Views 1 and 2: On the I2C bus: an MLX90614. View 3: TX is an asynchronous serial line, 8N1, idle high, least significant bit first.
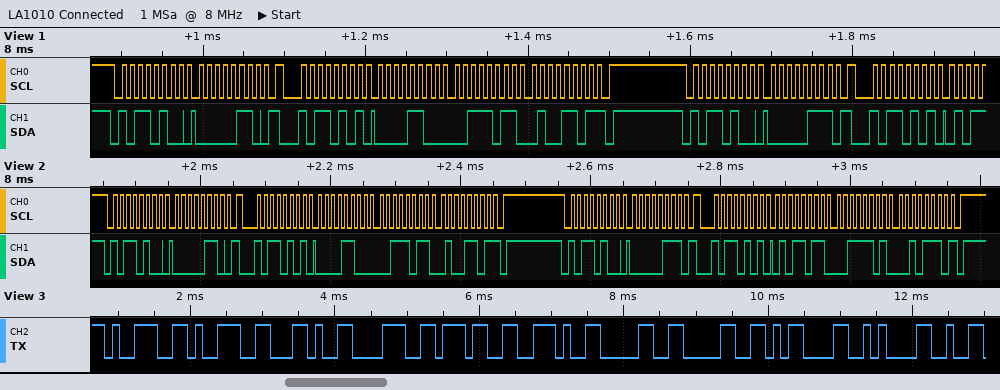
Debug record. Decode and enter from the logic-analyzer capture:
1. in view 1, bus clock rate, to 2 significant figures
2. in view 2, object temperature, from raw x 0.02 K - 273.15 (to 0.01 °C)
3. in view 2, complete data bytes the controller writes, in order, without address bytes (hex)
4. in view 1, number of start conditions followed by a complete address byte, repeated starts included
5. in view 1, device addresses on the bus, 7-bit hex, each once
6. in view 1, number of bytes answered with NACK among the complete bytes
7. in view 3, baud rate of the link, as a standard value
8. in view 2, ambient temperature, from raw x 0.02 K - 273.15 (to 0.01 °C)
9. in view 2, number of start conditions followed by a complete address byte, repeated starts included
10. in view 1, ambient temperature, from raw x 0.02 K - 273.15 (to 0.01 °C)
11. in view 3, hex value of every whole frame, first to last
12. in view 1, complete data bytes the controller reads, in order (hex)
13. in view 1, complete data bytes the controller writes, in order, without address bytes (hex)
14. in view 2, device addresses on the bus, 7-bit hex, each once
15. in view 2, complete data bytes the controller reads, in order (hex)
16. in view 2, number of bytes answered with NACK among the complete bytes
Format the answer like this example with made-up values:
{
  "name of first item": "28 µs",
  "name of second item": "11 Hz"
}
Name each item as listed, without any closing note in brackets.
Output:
{
  "in view 1, bus clock rate, to 2 significant figures": "100 kHz",
  "in view 2, object temperature, from raw x 0.02 K - 273.15": "40.99 °C",
  "in view 2, complete data bytes the controller writes, in order, without address bytes": "06 07",
  "in view 1, number of start conditions followed by a complete address byte, repeated starts included": "4",
  "in view 1, device addresses on the bus, 7-bit hex, each once": "0x5A",
  "in view 1, number of bytes answered with NACK among the complete bytes": "1",
  "in view 3, baud rate of the link, as a standard value": "9600 baud",
  "in view 2, ambient temperature, from raw x 0.02 K - 273.15": "29.17 °C",
  "in view 2, number of start conditions followed by a complete address byte, repeated starts included": "4",
  "in view 1, ambient temperature, from raw x 0.02 K - 273.15": "29.17 °C",
  "in view 3, hex value of every whole frame, first to last": "39 39 2C 38 37 2E 30 30 0D 0A",
  "in view 1, complete data bytes the controller reads, in order": "0C 3B 4D",
  "in view 1, complete data bytes the controller writes, in order, without address bytes": "06 07",
  "in view 2, device addresses on the bus, 7-bit hex, each once": "0x5A",
  "in view 2, complete data bytes the controller reads, in order": "0C 3B 4D 5B 3D 2E",
  "in view 2, number of bytes answered with NACK among the complete bytes": "2"
}
